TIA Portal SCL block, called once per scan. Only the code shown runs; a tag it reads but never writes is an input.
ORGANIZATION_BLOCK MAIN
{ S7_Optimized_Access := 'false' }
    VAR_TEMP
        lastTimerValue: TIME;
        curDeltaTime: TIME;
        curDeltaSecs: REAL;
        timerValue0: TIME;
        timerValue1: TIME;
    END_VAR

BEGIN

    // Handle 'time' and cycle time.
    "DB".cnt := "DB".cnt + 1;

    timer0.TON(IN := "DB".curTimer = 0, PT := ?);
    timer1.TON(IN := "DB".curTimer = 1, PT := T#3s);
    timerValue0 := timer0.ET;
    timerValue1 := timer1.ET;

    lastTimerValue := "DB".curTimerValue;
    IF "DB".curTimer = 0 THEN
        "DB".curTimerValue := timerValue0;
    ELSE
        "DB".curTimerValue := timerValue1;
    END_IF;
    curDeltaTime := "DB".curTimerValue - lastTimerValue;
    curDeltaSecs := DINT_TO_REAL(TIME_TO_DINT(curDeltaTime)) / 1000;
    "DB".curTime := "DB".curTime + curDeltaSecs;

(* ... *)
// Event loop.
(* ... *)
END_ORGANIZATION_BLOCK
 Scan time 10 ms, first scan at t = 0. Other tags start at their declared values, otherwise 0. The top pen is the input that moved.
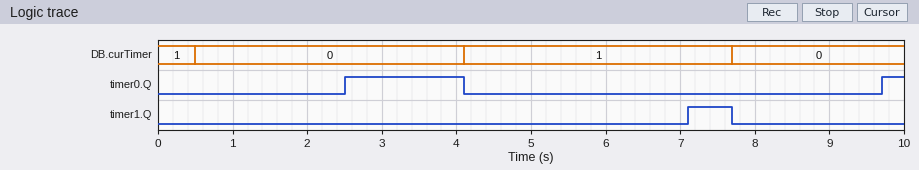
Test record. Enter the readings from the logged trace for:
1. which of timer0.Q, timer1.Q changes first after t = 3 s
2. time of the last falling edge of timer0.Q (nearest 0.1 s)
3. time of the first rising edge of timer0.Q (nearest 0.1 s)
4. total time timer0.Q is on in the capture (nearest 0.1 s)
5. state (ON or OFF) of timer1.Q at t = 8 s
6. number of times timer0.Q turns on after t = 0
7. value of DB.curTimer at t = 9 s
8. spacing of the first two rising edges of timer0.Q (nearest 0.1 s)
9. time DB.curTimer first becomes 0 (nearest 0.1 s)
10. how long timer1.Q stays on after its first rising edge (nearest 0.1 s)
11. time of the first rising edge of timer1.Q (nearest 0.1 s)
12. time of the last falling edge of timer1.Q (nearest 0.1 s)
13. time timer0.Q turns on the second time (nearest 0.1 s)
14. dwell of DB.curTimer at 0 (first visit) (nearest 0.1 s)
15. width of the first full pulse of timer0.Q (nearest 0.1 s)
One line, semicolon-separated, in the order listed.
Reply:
timer0.Q; 4.1 s; 2.5 s; 1.9 s; OFF; 2; 0; 7.2 s; 0.5 s; 0.6 s; 7.1 s; 7.7 s; 9.7 s; 3.6 s; 1.6 s
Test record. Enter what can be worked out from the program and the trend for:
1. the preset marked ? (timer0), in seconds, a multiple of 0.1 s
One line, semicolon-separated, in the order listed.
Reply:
2.0 s
